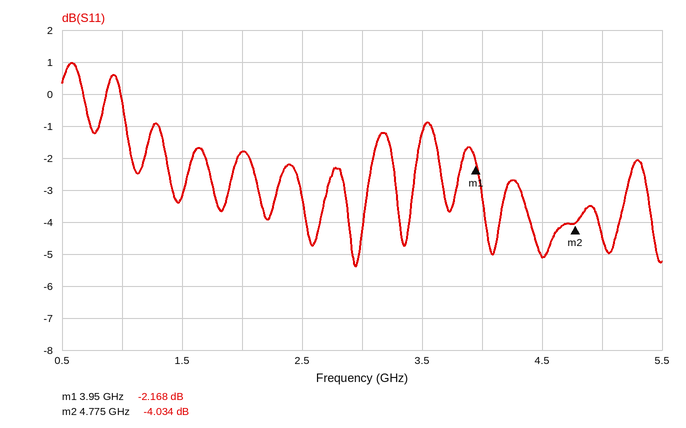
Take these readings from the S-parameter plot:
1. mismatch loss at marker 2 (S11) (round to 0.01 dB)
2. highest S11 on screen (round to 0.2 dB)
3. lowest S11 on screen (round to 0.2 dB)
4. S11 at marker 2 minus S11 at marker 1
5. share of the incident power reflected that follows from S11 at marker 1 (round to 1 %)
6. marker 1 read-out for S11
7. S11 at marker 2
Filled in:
2.18 dB
1.0 dB
-5.4 dB
-1.866 dB
61 %
-2.168 dB
-4.034 dB
